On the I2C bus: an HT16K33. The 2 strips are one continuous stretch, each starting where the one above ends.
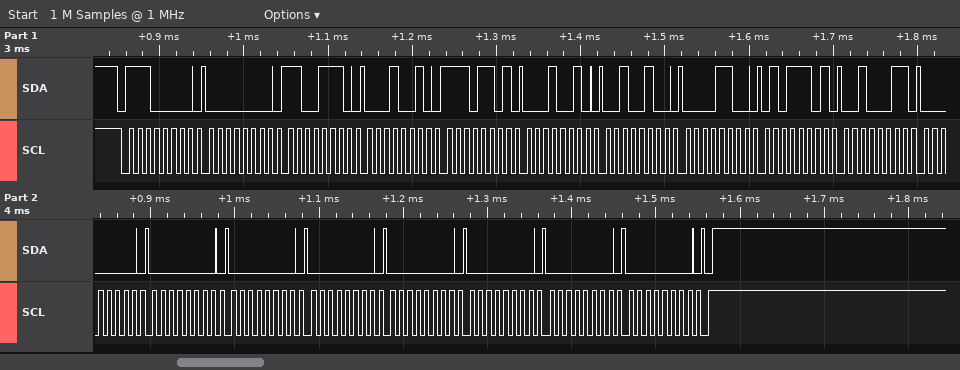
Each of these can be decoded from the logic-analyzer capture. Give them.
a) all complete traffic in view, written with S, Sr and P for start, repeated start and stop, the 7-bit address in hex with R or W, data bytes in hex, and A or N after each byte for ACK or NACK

S 70W A 00 A CE A 12 A ED A 12 A 24 A 0C A 5D A 23 A 00 A 00 A 00 A 00 A 00 A 00 A 00 A 00 A P
